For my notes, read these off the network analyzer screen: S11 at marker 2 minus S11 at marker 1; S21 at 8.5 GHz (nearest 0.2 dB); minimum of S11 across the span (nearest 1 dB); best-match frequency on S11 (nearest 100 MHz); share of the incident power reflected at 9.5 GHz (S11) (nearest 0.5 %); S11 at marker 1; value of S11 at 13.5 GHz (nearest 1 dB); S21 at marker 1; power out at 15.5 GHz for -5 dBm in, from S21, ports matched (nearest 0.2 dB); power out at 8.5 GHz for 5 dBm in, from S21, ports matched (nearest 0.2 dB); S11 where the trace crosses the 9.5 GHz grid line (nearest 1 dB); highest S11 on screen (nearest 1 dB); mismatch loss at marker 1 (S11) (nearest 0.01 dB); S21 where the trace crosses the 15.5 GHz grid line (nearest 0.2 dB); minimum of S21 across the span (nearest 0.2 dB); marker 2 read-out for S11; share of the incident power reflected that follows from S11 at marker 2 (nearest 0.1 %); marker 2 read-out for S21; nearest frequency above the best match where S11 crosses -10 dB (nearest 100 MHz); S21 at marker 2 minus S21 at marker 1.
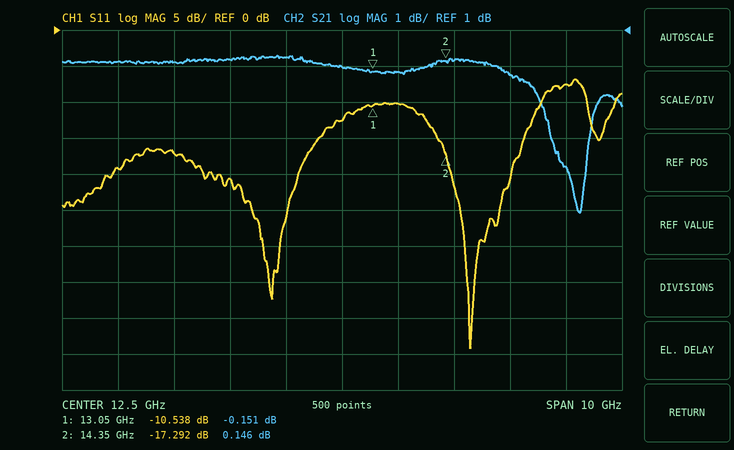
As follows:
-6.754 dB
0.2 dB
-44 dB
14.8 GHz
2.0 %
-10.538 dB
-10 dB
-0.151 dB
-5.2 dBm
5.2 dBm
-17 dB
-7 dB
0.40 dB
-0.2 dB
-4.0 dB
-17.292 dB
1.9 %
0.146 dB
16.1 GHz
0.297 dB
